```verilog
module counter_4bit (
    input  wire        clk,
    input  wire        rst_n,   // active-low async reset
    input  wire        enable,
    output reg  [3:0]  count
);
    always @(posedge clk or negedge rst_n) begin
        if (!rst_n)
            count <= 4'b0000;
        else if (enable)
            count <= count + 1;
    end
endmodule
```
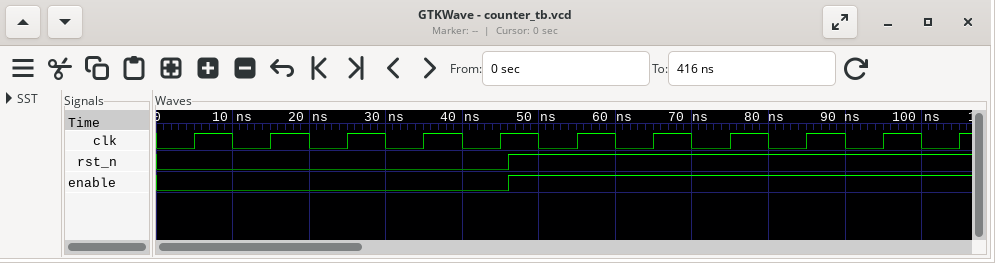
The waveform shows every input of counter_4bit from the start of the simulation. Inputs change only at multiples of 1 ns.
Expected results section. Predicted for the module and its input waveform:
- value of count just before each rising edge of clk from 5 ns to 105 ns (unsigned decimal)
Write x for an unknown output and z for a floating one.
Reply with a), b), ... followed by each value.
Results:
a) 0, 0, 0, 0, 0, 0, 1, 2, 3, 4, 5
